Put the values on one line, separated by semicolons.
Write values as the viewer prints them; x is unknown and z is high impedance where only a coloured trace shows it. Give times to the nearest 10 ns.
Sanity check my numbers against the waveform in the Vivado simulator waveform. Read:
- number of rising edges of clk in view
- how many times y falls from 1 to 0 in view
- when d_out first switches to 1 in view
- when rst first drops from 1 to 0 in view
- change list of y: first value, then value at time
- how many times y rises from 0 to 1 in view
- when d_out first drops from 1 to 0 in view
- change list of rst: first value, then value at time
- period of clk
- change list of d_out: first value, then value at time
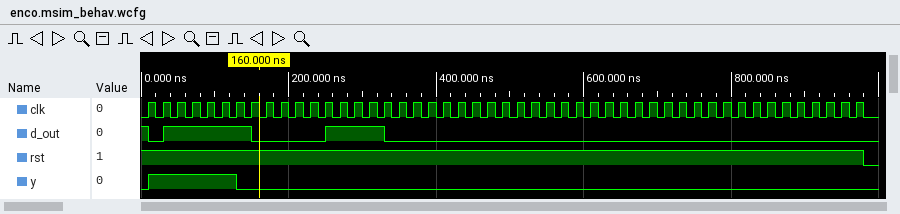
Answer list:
49; 1; 30 ns; 980 ns; 0, 1 at 10 ns, 0 at 130 ns; 1; 10 ns; 1, 0 at 980 ns; 20 ns; 1, 0 at 10 ns, 1 at 30 ns, 0 at 150 ns, 1 at 250 ns, 0 at 330 ns
